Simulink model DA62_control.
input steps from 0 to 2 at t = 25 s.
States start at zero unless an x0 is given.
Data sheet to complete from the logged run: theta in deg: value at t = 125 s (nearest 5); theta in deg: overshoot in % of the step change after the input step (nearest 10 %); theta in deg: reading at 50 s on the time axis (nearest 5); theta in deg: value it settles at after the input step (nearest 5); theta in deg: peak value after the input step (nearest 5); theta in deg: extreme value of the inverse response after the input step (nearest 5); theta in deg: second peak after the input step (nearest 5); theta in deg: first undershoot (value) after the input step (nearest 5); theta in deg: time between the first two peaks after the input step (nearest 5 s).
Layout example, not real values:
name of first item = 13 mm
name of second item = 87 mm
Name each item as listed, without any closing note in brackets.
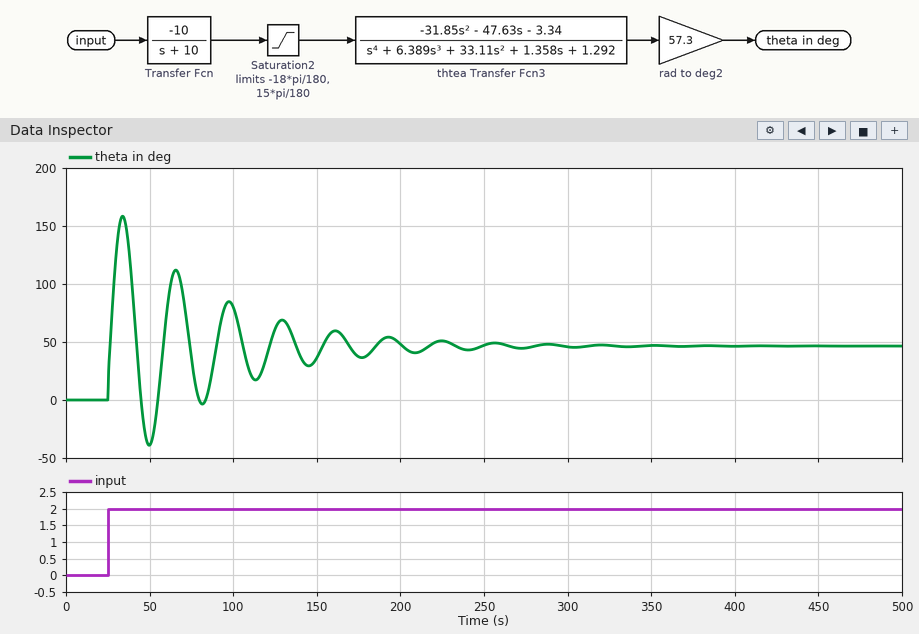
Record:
theta in deg: value at t = 125 s = 60
theta in deg: overshoot in % of the step change after the input step = 240 %
theta in deg: reading at 50 s on the time axis = -40
theta in deg: value it settles at after the input step = 45
theta in deg: peak value after the input step = 160
theta in deg: extreme value of the inverse response after the input step = -40
theta in deg: second peak after the input step = 110
theta in deg: first undershoot (value) after the input step = -40
theta in deg: time between the first two peaks after the input step = 30 s
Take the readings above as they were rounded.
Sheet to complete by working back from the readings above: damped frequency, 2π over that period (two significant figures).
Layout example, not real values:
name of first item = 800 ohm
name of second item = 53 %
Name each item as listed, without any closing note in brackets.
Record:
damped frequency, 2π over that period = 0.21 rad/s
